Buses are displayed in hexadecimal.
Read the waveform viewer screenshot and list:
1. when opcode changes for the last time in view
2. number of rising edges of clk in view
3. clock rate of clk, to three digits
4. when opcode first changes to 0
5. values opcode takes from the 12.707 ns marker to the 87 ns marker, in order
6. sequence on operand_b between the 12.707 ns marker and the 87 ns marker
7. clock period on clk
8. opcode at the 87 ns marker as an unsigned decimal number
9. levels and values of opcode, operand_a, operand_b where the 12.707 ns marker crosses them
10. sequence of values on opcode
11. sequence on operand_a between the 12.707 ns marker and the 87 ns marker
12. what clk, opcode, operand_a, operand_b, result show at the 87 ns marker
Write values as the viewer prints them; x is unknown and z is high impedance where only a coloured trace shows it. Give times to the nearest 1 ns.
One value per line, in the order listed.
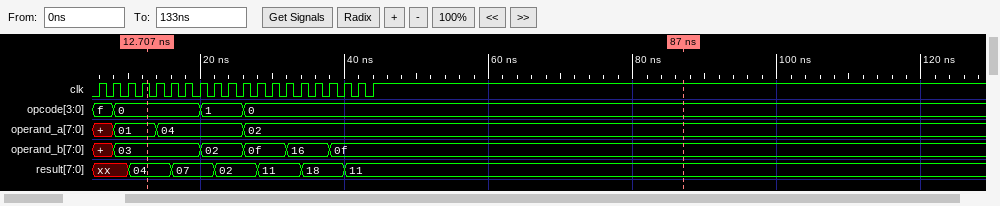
26 ns
20
500 MHz
8 ns
0, 1, 0
03, 02, 0f, 16, 0f
2 ns
0
opcode=0, operand_a=01, operand_b=03
f, 0, 1, 0
01, 04, 02
clk=1, opcode=0, operand_a=02, operand_b=0f, result=11
